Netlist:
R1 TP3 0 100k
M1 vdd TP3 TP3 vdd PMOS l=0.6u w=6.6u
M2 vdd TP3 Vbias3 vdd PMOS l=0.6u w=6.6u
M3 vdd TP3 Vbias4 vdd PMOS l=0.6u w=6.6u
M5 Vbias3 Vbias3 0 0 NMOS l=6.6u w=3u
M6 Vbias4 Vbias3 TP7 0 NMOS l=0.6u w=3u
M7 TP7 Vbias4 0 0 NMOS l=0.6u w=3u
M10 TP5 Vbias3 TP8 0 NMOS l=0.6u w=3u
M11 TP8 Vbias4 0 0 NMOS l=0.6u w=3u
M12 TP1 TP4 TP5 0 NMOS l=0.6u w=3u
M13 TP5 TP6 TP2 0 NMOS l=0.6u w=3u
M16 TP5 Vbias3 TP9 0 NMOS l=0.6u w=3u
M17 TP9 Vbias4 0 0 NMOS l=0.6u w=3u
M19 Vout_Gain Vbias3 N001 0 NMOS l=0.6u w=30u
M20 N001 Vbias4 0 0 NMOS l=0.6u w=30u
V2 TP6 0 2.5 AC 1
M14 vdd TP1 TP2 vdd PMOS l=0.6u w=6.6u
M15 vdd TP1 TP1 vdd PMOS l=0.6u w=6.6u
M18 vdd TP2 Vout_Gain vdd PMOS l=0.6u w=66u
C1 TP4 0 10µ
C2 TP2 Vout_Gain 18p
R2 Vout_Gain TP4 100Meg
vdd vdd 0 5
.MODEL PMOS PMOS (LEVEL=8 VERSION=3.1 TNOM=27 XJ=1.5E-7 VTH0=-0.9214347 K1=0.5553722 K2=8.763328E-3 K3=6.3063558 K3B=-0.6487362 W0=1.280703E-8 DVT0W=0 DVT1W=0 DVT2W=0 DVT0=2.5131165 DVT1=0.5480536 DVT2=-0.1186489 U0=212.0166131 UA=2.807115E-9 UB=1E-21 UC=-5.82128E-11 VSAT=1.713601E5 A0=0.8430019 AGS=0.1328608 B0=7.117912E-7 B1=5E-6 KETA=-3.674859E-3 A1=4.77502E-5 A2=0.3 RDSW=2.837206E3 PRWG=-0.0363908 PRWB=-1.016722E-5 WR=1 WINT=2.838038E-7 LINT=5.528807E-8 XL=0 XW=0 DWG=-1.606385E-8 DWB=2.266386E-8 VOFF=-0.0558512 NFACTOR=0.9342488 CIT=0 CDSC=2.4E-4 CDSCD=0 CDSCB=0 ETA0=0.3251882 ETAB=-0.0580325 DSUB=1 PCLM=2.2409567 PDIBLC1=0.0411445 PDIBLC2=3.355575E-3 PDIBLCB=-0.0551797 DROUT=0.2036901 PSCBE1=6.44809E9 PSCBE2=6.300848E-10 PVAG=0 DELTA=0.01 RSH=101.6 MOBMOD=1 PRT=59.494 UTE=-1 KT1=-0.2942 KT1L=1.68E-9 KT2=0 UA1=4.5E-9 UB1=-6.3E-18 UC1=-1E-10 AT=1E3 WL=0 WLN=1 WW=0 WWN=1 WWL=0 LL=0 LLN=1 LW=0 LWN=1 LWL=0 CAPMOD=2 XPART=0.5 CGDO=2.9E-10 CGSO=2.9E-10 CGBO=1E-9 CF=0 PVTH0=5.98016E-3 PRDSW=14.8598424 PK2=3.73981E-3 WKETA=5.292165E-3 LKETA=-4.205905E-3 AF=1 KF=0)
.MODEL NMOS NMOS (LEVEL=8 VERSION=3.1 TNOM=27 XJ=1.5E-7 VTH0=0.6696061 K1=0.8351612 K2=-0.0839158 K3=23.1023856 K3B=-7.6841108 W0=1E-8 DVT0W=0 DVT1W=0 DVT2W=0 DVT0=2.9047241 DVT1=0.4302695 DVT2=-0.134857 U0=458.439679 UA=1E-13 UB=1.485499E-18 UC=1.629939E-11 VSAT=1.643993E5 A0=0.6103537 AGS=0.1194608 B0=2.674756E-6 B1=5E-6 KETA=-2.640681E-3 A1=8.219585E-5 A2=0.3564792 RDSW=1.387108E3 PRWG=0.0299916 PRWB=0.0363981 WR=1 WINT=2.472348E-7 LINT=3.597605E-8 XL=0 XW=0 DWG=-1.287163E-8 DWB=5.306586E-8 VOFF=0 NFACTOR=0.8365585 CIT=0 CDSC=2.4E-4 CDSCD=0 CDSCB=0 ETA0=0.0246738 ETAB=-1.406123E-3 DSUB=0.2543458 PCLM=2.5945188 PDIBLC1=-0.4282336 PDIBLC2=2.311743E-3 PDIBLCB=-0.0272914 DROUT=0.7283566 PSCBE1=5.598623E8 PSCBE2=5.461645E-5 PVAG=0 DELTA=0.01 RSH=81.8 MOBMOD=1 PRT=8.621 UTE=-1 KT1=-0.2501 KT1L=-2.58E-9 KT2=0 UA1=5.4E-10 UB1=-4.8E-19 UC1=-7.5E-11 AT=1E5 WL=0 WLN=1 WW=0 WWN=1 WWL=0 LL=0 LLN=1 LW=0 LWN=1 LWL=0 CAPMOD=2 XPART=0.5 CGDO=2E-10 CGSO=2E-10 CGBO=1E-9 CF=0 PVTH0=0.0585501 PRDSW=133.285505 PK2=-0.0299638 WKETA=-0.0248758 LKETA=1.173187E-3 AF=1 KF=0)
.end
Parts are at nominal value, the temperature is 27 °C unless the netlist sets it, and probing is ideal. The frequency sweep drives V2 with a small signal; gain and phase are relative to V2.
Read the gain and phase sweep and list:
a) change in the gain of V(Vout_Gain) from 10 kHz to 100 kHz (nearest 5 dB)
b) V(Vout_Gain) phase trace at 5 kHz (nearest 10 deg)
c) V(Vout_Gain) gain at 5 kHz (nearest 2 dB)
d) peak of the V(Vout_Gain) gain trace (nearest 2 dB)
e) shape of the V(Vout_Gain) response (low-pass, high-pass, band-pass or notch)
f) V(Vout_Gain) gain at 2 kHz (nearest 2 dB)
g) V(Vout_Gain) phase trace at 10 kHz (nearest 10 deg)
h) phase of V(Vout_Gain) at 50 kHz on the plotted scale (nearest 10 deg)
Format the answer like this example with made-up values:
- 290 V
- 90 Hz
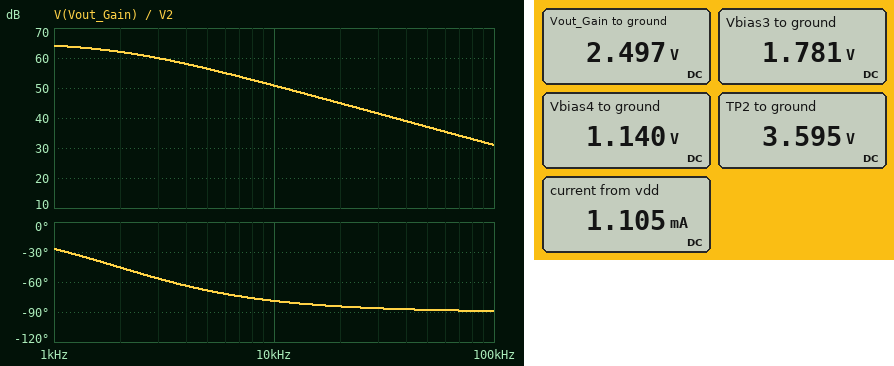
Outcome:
- -20 dB
- -70 deg
- 56 dB
- 64 dB
- low-pass
- 62 dB
- -80 deg
- -90 deg
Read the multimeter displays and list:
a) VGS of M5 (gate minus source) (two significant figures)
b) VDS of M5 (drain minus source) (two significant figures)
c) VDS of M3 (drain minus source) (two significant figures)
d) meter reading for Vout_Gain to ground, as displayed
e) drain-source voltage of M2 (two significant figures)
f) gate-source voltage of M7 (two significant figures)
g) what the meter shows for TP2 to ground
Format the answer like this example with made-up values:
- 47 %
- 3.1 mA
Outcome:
- 1.8 V
- 1.8 V
- 3.9 V
- 2.497 V
- 3.2 V
- 1.1 V
- 3.595 V
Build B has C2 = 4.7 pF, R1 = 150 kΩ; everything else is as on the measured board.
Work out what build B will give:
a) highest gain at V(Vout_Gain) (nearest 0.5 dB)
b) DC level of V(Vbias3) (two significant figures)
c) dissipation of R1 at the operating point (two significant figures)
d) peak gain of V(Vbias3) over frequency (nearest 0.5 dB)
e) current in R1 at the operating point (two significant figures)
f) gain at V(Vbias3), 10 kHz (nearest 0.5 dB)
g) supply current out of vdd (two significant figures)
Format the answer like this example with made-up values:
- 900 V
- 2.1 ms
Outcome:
- 68.0 dB
- 1.6 V
- 95 µW
- -40.5 dB
- 25 µA
- -41.5 dB
- 830 µA
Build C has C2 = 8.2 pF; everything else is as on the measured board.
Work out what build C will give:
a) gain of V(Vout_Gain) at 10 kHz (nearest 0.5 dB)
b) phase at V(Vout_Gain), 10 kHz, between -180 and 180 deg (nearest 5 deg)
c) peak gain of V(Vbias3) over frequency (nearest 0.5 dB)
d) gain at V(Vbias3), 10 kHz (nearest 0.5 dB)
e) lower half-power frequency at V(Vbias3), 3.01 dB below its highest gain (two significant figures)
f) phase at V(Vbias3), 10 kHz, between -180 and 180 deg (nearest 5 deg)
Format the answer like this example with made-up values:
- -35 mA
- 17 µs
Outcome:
- 57.0 dB
- -65 deg
- -45.5 dB
- -46.0 dB
- 4.3 kHz
- 25 deg
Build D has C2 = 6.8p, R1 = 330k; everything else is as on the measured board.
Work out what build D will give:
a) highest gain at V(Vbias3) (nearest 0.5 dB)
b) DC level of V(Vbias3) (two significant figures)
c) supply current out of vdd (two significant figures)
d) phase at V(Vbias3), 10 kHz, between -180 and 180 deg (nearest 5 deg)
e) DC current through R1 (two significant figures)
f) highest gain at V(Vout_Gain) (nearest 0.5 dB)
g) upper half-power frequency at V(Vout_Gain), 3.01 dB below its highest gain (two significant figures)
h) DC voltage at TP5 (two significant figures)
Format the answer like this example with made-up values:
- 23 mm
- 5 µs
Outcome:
- -45.0 dB
- 1.3 V
- 470 µA
- 10 deg
- 12 µA
- 71.0 dB
- 1.8 kHz
- 1.2 V
